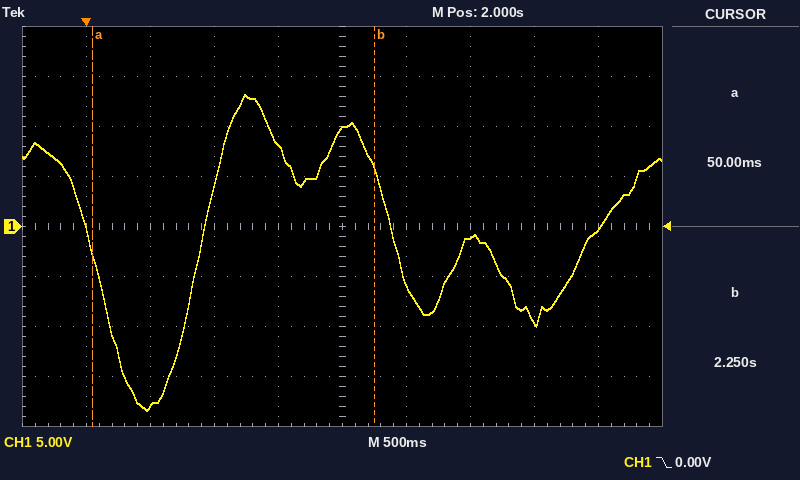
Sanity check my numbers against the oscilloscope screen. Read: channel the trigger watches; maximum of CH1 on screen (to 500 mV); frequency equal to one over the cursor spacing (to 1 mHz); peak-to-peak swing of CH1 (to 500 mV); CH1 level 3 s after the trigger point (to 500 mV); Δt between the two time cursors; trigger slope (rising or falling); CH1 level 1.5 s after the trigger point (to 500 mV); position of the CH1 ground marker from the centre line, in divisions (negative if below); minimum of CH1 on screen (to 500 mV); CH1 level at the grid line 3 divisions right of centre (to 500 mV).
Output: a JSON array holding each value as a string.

["CH1", "13.0 V", "455 mHz", "31.5 V", "-1.0 V", "2.20 s", "falling", "8.0 V", "0.0 div", "-18.5 V", "-9.5 V"]
